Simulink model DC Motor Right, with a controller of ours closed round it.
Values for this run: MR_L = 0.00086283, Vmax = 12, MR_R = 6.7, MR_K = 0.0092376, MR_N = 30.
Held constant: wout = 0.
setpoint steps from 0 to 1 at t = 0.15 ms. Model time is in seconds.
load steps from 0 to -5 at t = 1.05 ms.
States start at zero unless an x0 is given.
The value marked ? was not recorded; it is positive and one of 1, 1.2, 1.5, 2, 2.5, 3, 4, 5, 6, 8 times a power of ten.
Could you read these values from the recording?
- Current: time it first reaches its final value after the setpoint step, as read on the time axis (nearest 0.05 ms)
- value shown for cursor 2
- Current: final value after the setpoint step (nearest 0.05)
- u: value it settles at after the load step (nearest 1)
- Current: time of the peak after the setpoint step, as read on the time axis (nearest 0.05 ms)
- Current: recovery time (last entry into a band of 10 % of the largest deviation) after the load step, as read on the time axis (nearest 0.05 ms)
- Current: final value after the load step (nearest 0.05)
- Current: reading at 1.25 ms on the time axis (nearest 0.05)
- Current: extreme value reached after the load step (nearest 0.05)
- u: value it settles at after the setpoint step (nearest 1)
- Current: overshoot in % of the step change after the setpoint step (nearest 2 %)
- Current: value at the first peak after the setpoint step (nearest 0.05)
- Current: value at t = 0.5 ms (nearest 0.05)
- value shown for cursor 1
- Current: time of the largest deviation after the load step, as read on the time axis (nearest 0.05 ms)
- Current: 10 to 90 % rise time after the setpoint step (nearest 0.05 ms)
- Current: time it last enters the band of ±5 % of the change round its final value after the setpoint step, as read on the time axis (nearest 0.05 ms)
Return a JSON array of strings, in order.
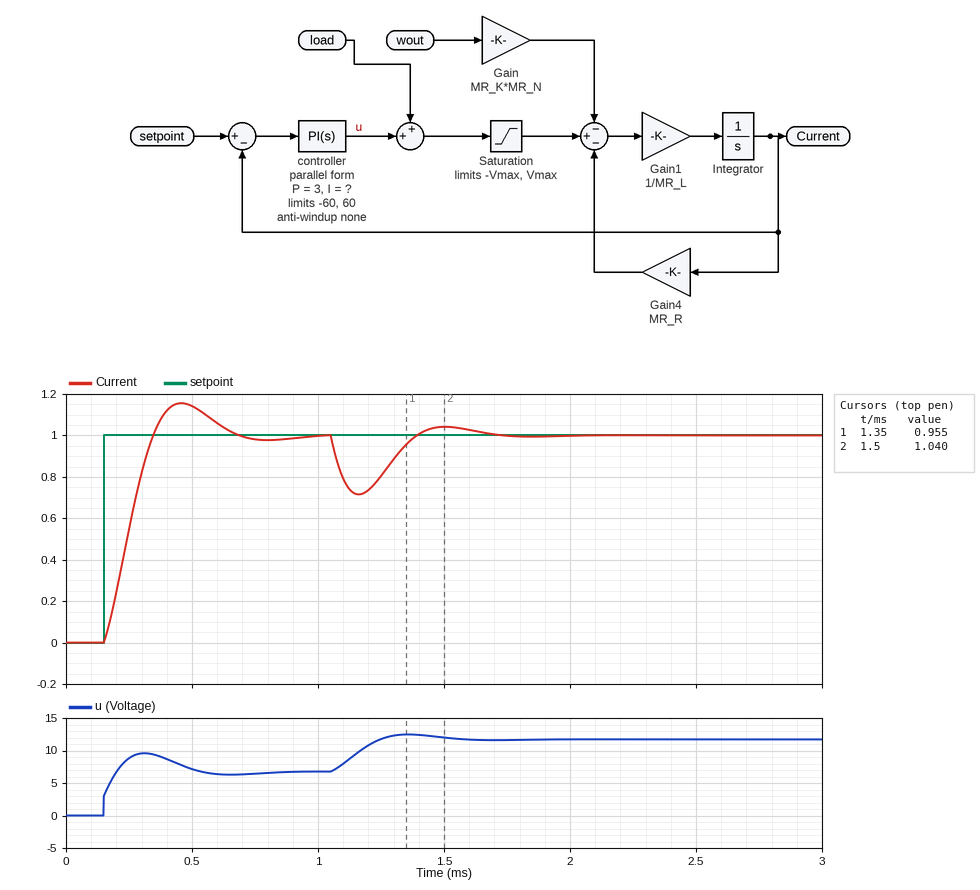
["0.35 ms", "1.040", "1.00", "12", "0.45 ms", "1.60 ms", "1.00", "0.80", "0.70", "7", "16 %", "1.15", "1.15", "0.955", "1.15 ms", "0.15 ms", "0.60 ms"]
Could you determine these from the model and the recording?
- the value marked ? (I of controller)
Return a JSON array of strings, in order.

["100000"]
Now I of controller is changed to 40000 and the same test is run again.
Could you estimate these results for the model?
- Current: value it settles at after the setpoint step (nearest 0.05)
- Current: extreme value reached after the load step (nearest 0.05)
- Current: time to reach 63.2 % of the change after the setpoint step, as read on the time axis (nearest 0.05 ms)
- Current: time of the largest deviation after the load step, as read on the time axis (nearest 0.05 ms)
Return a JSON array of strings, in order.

["1.00", "0.65", "0.35 ms", "1.20 ms"]
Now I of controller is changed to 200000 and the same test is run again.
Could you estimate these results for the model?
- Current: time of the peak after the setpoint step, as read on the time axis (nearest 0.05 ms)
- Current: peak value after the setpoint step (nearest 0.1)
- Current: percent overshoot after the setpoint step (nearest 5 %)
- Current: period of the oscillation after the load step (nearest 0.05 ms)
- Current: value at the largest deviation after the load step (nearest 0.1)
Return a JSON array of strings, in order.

["0.35 ms", "1.3", "30 %", "0.45 ms", "0.8"]
